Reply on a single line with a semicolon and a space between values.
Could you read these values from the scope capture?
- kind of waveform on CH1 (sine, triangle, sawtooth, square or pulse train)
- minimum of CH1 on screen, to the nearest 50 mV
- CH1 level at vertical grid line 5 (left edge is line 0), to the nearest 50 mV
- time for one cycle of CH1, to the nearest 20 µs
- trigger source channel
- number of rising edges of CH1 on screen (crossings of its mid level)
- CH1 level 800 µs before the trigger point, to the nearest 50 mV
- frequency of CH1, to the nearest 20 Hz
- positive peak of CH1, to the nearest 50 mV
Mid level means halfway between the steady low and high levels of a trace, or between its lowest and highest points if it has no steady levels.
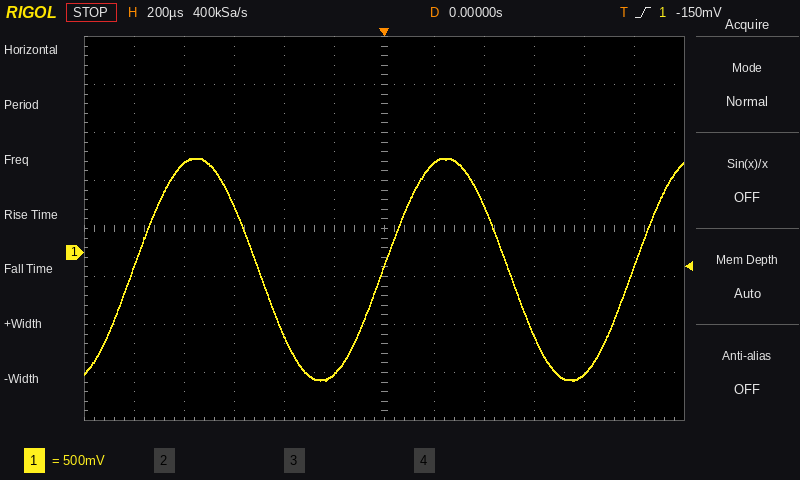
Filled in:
sine; -1.35 V; -1.25 V; 1.00 ms; CH1; 3; 950 mV; 1.00 kHz; 1.00 V
